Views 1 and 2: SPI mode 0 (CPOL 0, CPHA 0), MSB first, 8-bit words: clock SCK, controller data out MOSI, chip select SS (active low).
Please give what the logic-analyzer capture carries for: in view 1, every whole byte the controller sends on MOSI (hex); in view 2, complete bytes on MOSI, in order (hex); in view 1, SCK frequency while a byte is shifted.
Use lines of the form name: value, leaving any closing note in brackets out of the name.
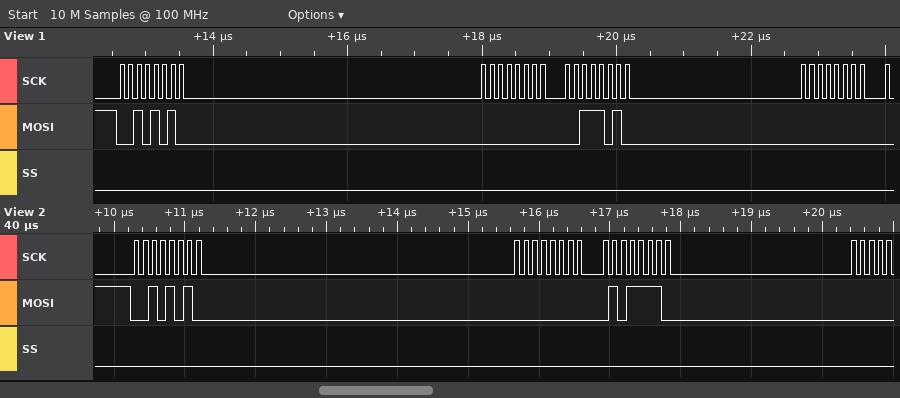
in view 1, every whole byte the controller sends on MOSI: 0x2A 0x00 0x3A 0x00
in view 2, complete bytes on MOSI, in order: 2A 00 5E
in view 1, SCK frequency while a byte is shifted: 8 MHz
